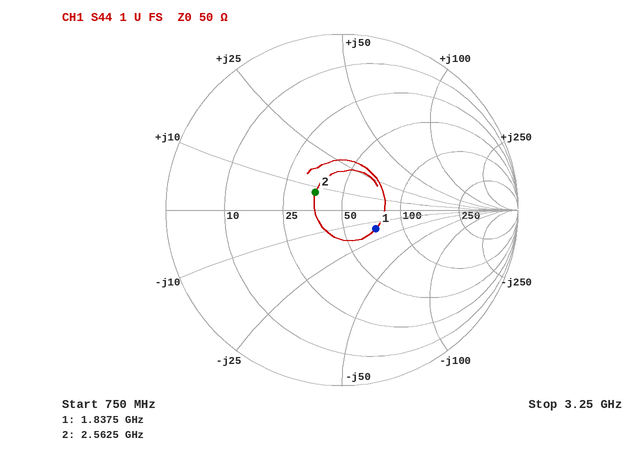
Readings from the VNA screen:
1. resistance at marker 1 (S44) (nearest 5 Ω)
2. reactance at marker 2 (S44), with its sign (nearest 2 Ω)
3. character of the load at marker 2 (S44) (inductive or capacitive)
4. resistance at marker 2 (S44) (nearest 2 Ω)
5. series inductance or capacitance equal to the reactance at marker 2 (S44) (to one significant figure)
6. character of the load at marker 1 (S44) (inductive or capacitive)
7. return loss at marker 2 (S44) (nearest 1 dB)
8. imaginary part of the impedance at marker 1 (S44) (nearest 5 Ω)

70 Ω
+8 Ω
inductive
36 Ω
500 pH
capacitive
15 dB
-15 Ω
